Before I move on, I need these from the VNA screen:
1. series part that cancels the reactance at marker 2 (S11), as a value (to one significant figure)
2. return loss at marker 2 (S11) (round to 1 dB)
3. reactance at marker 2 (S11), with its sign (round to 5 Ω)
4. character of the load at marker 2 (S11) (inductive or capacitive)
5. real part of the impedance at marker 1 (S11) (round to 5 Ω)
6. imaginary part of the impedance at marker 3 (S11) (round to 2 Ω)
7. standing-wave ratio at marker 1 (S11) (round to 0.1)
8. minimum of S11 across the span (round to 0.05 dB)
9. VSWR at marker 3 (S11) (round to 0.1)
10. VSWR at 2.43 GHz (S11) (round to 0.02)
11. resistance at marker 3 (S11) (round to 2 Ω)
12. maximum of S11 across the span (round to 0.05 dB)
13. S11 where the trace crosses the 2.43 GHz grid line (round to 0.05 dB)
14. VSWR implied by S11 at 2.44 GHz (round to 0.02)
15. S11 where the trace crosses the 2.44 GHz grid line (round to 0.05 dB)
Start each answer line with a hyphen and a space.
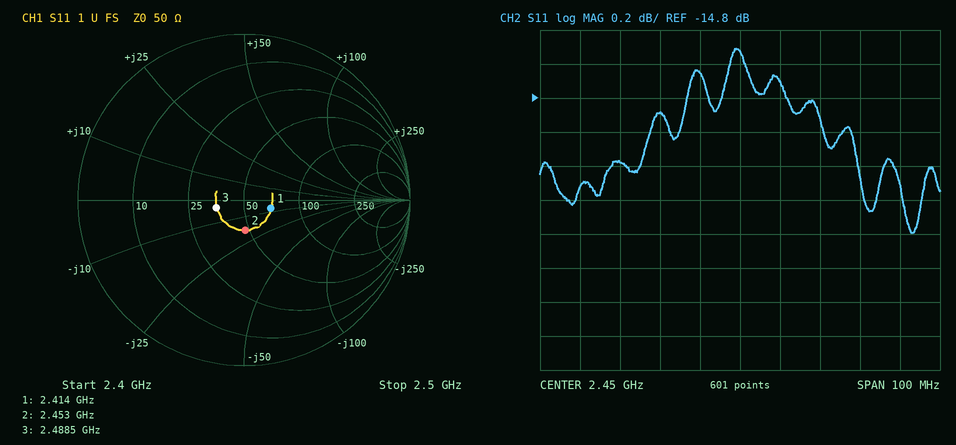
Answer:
- 1 nH
- 15 dB
- -20 Ω
- capacitive
- 70 Ω
- -4 Ω
- 1.4
- -15.60 dB
- 1.4
- 1.44
- 36 Ω
- -14.50 dB
- -14.90 dB
- 1.46
- -14.65 dB
